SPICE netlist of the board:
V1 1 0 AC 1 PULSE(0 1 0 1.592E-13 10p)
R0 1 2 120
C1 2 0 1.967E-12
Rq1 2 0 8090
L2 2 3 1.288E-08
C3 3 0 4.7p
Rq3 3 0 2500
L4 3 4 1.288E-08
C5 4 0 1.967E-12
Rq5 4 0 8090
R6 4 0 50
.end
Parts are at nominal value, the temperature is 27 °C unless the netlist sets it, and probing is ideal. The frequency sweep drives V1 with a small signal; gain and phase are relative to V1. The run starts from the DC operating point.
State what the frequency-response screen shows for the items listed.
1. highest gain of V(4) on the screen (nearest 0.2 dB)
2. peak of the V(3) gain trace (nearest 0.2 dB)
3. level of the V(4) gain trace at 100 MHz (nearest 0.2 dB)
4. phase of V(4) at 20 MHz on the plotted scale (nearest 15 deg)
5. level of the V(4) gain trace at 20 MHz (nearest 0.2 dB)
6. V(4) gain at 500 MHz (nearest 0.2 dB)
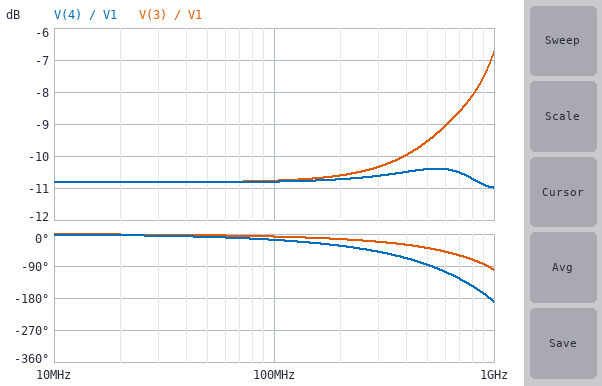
-10.4 dB
-6.8 dB
-10.8 dB
0 deg
-10.8 dB
-10.4 dB
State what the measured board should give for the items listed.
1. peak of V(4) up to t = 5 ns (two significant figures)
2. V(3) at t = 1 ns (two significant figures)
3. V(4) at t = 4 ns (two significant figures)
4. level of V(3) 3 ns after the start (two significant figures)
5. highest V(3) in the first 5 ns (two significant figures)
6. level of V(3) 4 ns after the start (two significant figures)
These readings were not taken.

340 mV
240 mV
290 mV
290 mV
390 mV
290 mV
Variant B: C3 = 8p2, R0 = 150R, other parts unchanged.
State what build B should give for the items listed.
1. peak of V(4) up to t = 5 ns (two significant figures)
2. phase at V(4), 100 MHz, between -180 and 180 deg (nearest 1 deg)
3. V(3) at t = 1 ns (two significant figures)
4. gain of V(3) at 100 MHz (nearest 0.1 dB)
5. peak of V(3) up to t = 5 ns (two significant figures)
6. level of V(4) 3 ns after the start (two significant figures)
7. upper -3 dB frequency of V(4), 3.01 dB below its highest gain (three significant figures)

260 mV
-21 deg
230 mV
-12.3 dB
280 mV
240 mV
1.06 GHz
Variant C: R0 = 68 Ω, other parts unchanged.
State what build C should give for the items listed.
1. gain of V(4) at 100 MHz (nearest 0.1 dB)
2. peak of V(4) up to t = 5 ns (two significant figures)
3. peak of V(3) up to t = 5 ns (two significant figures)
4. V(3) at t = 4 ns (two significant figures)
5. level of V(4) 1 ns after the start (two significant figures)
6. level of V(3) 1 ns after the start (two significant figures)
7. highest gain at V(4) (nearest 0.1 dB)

-7.6 dB
480 mV
540 mV
420 mV
460 mV
360 mV
-7.5 dB
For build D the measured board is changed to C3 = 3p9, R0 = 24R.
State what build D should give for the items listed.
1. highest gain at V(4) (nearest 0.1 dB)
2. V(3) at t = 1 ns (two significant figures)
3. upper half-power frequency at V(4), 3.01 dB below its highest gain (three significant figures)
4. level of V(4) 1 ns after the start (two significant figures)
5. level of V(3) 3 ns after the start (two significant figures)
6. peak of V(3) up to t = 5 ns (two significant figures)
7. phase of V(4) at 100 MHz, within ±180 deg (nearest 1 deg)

-3.5 dB
560 mV
1.20 GHz
690 mV
670 mV
820 mV
-17 deg
